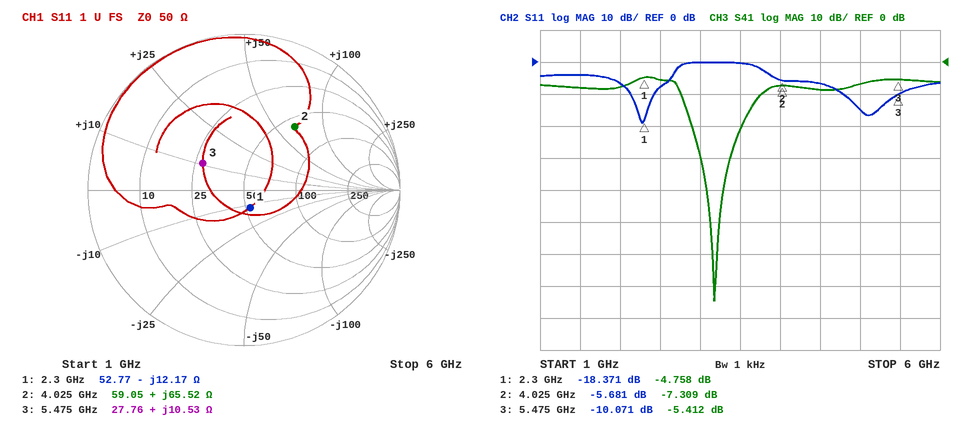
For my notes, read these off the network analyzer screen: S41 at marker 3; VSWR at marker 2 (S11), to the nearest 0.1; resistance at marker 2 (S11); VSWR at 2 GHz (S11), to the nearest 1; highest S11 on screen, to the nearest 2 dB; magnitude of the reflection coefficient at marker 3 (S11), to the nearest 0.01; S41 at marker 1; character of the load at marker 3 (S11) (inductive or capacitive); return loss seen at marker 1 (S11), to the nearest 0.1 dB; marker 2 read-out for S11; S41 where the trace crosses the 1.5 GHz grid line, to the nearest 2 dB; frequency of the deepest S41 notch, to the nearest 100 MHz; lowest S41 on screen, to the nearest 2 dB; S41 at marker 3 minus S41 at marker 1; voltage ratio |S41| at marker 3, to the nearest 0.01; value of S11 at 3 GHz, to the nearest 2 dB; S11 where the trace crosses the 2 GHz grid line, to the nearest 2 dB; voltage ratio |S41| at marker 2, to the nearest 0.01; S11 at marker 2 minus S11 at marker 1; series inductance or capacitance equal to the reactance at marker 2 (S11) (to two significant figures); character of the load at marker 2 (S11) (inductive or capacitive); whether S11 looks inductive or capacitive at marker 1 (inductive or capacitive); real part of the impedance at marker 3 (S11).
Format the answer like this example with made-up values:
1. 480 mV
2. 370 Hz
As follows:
1. -5.412 dB
2. 3.2
3. 59.05 Ω
4. 3
5. 0 dB
6. 0.31
7. -4.758 dB
8. inductive
9. 18.4 dB
10. -5.681 dB
11. -8 dB
12. 3.2 GHz
13. -74 dB
14. -0.654 dB
15. 0.54
16. 0 dB
17. -6 dB
18. 0.43
19. 12.690 dB
20. 2.6 nH
21. inductive
22. capacitive
23. 27.76 Ω
